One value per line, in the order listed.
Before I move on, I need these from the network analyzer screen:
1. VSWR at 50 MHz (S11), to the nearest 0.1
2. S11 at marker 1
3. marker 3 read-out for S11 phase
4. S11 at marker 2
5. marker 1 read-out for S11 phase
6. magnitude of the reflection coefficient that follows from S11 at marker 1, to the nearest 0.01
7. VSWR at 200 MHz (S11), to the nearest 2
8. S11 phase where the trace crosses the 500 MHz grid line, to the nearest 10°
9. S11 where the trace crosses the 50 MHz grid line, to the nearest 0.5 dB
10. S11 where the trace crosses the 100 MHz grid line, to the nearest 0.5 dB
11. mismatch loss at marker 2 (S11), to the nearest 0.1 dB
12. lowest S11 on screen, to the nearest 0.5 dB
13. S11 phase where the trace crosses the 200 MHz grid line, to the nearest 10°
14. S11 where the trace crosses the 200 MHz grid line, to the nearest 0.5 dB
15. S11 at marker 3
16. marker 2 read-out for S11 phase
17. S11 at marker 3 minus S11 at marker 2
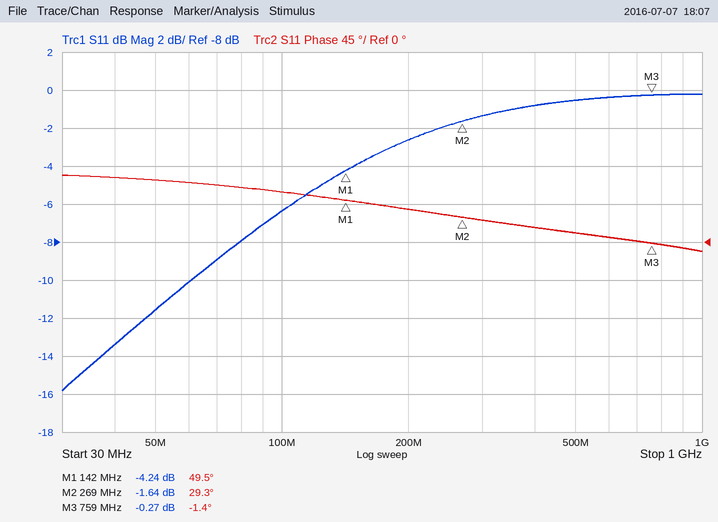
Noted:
1.7
-4.24 dB
-1.4°
-1.64 dB
49.5°
0.61
6
10°
-11.5 dB
-6.5 dB
5.0 dB
-16.0 dB
40°
-2.5 dB
-0.27 dB
29.3°
1.37 dB
